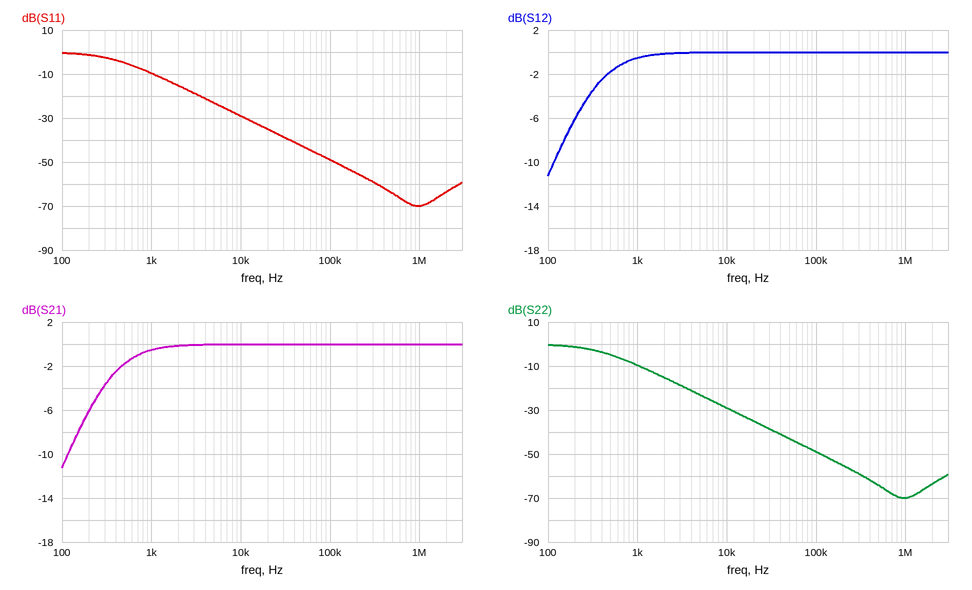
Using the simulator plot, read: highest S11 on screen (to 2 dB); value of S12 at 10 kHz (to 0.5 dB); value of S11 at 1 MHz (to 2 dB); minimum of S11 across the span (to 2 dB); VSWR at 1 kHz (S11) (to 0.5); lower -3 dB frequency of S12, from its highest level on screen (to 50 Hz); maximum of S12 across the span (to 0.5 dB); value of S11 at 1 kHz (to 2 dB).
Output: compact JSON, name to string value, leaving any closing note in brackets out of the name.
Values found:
{"highest S11 on screen": "0 dB", "value of S12 at 10 kHz": "0.0 dB", "value of S11 at 1 MHz": "-70 dB", "minimum of S11 across the span": "-70 dB", "VSWR at 1 kHz (S11)": "2.0", "lower -3 dB frequency of S12, from its highest level on screen": "350 Hz", "maximum of S12 across the span": "0.0 dB", "value of S11 at 1 kHz": "-10 dB"}
